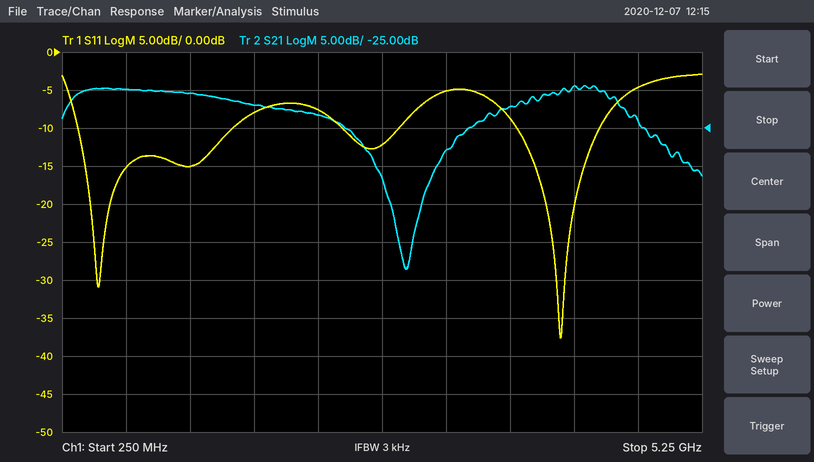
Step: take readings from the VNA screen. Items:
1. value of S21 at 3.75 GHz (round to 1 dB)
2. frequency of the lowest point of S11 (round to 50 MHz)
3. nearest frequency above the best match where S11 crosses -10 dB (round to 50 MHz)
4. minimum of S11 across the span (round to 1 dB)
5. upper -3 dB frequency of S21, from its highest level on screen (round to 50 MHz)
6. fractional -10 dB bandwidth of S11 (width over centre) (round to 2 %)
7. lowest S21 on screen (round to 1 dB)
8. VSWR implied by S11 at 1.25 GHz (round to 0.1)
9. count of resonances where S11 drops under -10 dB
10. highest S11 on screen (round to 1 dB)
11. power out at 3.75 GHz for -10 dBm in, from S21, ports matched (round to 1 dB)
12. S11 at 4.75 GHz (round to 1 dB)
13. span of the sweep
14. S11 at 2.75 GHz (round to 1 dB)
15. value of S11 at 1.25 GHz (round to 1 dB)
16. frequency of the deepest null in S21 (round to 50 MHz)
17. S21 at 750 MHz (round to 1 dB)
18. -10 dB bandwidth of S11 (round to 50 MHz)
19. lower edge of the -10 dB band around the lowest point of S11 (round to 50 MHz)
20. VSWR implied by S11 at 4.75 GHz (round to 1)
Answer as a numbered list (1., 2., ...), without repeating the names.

1. -22 dB
2. 4.15 GHz
3. 4.45 GHz
4. -38 dB
5. 4.65 GHz
6. 16 %
7. -44 dB
8. 1.4
9. 3
10. -3 dB
11. -32 dBm
12. -5 dB
13. 5 GHz
14. -12 dB
15. -15 dB
16. 2.95 GHz
17. -20 dB
18. 650 MHz
19. 3.80 GHz
20. 4
